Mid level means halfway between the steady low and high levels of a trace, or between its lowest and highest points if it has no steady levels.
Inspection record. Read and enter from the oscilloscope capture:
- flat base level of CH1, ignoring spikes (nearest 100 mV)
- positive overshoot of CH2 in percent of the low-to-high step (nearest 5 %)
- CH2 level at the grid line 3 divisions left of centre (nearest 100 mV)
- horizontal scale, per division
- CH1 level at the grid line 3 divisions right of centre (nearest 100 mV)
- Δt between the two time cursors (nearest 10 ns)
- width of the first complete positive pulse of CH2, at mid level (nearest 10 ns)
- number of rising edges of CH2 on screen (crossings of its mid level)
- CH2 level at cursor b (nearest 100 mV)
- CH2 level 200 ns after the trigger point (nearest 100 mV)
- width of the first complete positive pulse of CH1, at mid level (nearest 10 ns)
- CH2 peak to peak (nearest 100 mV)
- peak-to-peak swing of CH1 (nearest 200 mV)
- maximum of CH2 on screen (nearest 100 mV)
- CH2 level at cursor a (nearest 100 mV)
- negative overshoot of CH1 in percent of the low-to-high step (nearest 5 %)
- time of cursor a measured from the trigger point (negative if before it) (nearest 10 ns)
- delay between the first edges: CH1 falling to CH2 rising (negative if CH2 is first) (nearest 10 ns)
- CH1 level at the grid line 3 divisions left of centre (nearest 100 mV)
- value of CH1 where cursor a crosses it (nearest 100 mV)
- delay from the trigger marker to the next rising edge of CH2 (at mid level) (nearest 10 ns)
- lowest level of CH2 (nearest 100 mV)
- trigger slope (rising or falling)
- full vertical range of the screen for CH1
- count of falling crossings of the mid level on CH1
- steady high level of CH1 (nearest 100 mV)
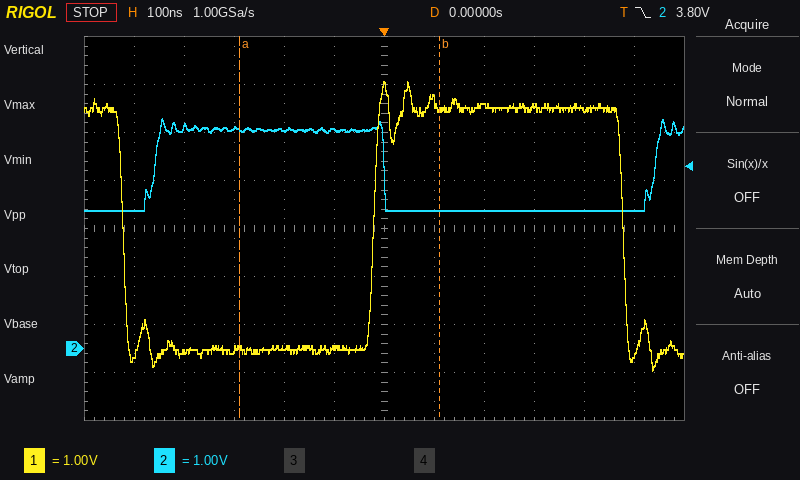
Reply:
0.0 V
15 %
4.6 V
100 ns
5.0 V
400 ns
460 ns
2
2.9 V
2.9 V
500 ns
1.9 V
6.0 V
4.8 V
4.6 V
10 %
-290 ns
+60 ns
0.0 V
0.0 V
540 ns
2.9 V
falling
8 V
2
5.0 V
